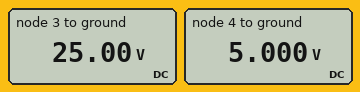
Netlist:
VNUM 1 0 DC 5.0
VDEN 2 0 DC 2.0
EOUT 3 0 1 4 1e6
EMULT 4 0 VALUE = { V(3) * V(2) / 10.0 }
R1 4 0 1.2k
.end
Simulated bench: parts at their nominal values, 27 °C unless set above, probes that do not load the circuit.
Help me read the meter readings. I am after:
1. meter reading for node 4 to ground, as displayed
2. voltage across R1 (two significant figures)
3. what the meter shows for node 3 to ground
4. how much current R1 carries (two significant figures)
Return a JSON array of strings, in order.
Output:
["5.000 V", "5.0 V", "25.00 V", "4.2 mA"]
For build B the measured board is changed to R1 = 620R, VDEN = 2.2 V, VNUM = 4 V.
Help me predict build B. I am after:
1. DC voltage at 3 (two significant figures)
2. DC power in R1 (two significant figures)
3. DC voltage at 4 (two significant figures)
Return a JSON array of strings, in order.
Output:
["18 V", "26 mW", "4.0 V"]
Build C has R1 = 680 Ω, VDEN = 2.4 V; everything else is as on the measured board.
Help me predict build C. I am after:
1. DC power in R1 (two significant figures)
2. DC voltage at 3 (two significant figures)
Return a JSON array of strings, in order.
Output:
["37 mW", "21 V"]
